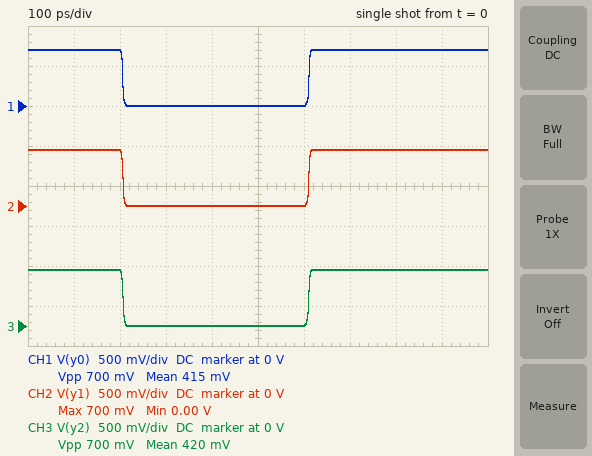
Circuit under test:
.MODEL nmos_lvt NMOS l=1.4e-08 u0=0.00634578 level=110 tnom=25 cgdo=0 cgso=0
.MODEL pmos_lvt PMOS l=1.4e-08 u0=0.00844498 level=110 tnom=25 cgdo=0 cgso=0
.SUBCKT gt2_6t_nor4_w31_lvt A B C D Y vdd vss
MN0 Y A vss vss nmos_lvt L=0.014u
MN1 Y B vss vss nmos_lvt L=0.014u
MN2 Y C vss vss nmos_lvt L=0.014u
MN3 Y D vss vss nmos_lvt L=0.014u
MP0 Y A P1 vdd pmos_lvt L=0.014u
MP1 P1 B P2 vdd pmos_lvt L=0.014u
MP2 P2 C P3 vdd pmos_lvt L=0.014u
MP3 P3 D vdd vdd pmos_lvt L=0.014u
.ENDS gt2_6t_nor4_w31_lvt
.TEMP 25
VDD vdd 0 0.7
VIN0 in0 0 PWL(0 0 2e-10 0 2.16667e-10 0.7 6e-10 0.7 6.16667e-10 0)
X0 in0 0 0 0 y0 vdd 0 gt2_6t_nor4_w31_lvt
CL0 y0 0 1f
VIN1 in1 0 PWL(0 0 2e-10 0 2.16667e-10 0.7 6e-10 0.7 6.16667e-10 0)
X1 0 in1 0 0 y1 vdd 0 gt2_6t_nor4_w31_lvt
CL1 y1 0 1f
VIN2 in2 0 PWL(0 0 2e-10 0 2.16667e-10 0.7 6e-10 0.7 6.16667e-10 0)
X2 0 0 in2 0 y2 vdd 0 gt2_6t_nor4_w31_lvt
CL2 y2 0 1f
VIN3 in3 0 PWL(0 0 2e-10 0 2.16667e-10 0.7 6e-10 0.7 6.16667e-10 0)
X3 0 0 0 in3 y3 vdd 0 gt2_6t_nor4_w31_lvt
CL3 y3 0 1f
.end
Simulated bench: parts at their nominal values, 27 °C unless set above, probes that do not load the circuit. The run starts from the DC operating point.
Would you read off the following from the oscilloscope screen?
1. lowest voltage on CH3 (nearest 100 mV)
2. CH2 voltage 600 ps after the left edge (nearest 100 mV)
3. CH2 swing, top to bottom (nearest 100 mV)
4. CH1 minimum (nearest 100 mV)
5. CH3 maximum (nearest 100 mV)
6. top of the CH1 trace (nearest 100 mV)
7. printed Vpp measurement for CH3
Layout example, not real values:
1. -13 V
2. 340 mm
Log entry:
1. 0 V
2. 0 V
3. 700 mV
4. 0 V
5. 700 mV
6. 700 mV
7. 700 mV
